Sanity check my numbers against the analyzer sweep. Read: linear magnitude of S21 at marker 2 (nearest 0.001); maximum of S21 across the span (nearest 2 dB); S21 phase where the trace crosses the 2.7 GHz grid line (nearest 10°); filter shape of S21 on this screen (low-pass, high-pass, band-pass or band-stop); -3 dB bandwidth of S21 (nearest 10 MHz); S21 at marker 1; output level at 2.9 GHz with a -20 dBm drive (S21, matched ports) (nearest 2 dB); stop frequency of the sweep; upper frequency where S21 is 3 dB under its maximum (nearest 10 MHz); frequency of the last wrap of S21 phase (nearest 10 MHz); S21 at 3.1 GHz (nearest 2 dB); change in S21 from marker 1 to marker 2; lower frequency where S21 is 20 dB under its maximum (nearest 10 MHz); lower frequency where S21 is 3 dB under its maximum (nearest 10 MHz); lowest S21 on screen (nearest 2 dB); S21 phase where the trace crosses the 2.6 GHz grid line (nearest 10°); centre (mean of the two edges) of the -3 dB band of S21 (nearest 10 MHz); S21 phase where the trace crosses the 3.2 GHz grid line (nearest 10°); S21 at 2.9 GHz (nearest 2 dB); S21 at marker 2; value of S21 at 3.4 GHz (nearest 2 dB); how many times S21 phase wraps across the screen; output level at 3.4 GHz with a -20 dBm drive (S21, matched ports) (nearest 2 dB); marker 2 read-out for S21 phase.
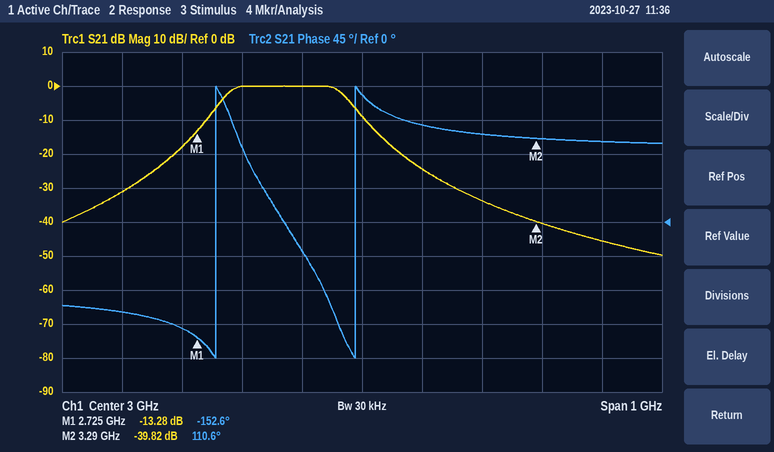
0.010
0 dB
-140°
band-pass
200 MHz
-13.28 dB
-20 dBm
3.5 GHz
2.97 GHz
2.99 GHz
-24 dB
-26.54 dB
2.69 GHz
2.77 GHz
-50 dB
-120°
2.87 GHz
120°
0 dB
-39.82 dB
-46 dB
2
-66 dBm
110.6°
